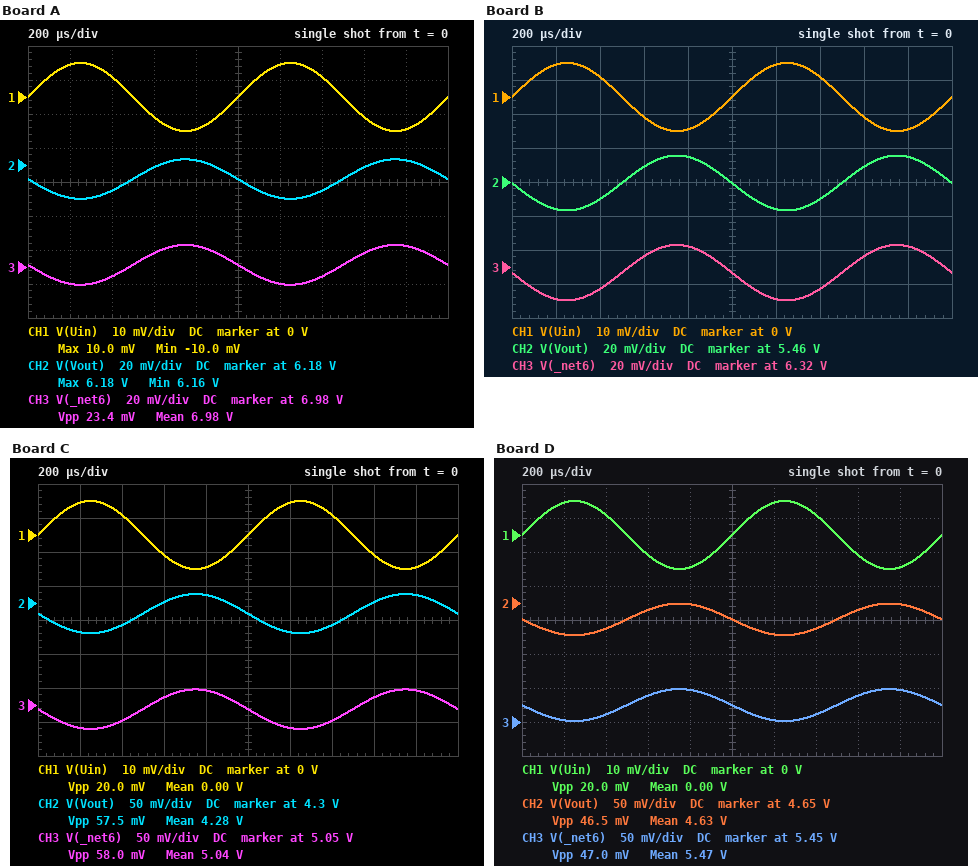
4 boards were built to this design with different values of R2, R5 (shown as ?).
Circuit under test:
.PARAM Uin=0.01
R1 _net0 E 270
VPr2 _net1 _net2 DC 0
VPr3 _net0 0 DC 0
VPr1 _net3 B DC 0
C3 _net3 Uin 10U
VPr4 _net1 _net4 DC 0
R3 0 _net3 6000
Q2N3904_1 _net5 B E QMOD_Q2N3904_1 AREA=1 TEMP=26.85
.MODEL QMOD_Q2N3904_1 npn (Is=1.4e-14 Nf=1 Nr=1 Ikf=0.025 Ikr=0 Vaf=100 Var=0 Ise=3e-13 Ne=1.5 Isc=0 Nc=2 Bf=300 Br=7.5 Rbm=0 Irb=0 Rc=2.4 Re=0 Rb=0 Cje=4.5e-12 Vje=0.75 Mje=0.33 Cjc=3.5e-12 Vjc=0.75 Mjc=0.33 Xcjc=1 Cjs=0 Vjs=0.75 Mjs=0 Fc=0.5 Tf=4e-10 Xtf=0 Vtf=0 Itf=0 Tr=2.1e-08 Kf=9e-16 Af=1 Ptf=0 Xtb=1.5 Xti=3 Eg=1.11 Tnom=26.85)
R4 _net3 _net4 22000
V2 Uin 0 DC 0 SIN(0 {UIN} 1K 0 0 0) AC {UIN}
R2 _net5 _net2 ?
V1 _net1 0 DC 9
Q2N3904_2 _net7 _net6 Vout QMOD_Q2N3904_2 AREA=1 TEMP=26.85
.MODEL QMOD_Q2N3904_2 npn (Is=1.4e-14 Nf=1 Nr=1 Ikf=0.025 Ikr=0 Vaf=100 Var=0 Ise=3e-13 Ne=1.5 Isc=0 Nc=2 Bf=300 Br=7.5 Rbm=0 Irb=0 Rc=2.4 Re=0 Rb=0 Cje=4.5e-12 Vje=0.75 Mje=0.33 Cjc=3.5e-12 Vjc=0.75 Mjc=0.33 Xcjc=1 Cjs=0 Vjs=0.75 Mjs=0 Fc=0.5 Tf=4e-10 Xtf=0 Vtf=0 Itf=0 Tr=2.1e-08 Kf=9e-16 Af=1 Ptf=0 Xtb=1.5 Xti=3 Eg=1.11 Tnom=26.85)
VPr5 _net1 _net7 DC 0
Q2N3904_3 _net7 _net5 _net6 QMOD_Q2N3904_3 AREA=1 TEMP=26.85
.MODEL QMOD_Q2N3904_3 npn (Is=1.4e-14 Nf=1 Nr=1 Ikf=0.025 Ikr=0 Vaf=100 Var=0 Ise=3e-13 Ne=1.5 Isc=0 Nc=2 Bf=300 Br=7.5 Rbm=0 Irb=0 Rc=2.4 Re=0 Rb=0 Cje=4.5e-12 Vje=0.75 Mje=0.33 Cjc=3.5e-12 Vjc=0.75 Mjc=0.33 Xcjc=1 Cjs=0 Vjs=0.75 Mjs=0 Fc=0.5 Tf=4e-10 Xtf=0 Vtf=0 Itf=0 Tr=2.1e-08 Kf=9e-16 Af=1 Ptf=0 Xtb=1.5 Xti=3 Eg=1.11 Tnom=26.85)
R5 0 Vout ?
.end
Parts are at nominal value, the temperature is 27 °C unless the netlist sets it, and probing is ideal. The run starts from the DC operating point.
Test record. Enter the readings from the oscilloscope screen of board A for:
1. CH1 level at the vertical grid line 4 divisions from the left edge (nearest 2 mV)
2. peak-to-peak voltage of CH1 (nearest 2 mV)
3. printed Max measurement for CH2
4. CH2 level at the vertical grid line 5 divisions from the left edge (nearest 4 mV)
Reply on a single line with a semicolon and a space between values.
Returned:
-10 mV; 20 mV; 6.18 V; 6.172 V
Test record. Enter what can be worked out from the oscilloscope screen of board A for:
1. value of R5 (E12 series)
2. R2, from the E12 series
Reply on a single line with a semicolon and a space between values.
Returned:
56 Ω; 330 Ω
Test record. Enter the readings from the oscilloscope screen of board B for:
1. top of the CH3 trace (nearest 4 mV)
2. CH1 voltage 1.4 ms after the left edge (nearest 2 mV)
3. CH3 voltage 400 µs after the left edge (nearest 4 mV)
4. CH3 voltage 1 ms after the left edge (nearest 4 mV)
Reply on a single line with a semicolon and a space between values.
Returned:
6.332 V; 6 mV; 6.308 V; 6.316 V
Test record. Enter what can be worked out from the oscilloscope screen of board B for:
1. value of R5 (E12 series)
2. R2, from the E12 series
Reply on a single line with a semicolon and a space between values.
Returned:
18 Ω; 470 Ω
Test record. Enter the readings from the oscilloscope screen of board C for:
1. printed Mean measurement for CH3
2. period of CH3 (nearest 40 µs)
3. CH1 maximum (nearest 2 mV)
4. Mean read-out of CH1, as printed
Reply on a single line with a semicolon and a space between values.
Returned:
5.04 V; 1.00 ms; 10 mV; 0.00 V
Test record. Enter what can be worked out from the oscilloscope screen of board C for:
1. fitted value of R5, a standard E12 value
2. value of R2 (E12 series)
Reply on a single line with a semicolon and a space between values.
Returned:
120 Ω; 820 Ω
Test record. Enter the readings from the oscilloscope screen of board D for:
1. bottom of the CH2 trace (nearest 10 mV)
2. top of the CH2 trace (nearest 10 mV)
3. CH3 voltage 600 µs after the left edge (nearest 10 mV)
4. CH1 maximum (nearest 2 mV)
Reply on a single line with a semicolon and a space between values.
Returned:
4.60 V; 4.65 V; 5.49 V; 10 mV
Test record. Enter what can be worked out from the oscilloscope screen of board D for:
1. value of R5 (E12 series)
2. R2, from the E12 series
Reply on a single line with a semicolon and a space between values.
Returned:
18 Ω; 680 Ω
